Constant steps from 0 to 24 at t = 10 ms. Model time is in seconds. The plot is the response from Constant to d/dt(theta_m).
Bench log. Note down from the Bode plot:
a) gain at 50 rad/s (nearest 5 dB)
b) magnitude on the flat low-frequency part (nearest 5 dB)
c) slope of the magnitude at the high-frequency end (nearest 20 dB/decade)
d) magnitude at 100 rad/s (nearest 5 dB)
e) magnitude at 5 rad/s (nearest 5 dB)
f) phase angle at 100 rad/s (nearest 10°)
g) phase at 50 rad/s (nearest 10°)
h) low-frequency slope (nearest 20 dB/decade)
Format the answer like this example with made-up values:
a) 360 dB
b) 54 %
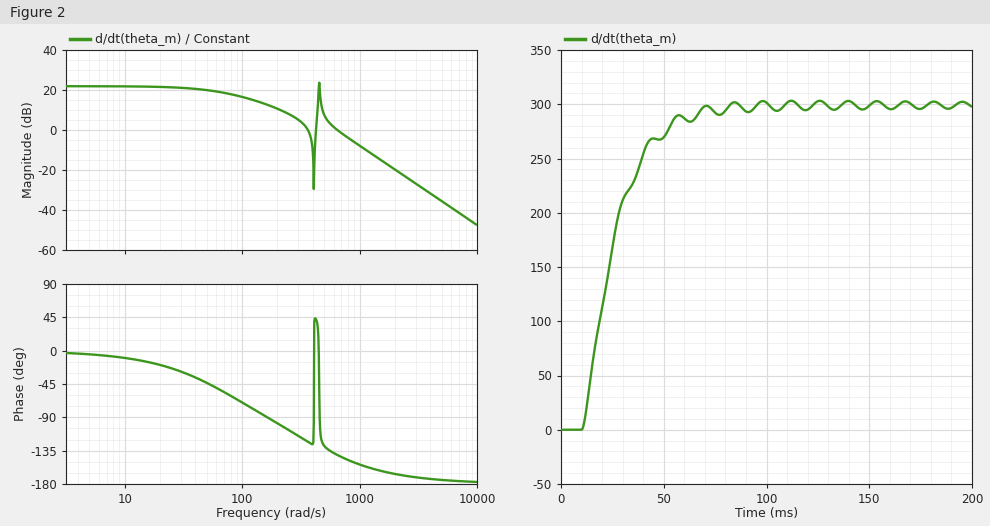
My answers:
a) 20 dB
b) 20 dB
c) -40 dB/decade
d) 15 dB
e) 20 dB
f) -70°
g) -40°
h) 0 dB/decade
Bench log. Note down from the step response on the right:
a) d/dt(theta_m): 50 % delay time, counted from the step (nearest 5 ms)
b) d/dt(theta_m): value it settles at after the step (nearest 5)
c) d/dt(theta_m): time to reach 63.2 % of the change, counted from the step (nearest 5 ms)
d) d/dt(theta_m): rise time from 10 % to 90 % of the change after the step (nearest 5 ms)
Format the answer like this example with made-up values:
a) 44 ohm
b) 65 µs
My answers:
a) 15 ms
b) 300
c) 15 ms
d) 35 ms
